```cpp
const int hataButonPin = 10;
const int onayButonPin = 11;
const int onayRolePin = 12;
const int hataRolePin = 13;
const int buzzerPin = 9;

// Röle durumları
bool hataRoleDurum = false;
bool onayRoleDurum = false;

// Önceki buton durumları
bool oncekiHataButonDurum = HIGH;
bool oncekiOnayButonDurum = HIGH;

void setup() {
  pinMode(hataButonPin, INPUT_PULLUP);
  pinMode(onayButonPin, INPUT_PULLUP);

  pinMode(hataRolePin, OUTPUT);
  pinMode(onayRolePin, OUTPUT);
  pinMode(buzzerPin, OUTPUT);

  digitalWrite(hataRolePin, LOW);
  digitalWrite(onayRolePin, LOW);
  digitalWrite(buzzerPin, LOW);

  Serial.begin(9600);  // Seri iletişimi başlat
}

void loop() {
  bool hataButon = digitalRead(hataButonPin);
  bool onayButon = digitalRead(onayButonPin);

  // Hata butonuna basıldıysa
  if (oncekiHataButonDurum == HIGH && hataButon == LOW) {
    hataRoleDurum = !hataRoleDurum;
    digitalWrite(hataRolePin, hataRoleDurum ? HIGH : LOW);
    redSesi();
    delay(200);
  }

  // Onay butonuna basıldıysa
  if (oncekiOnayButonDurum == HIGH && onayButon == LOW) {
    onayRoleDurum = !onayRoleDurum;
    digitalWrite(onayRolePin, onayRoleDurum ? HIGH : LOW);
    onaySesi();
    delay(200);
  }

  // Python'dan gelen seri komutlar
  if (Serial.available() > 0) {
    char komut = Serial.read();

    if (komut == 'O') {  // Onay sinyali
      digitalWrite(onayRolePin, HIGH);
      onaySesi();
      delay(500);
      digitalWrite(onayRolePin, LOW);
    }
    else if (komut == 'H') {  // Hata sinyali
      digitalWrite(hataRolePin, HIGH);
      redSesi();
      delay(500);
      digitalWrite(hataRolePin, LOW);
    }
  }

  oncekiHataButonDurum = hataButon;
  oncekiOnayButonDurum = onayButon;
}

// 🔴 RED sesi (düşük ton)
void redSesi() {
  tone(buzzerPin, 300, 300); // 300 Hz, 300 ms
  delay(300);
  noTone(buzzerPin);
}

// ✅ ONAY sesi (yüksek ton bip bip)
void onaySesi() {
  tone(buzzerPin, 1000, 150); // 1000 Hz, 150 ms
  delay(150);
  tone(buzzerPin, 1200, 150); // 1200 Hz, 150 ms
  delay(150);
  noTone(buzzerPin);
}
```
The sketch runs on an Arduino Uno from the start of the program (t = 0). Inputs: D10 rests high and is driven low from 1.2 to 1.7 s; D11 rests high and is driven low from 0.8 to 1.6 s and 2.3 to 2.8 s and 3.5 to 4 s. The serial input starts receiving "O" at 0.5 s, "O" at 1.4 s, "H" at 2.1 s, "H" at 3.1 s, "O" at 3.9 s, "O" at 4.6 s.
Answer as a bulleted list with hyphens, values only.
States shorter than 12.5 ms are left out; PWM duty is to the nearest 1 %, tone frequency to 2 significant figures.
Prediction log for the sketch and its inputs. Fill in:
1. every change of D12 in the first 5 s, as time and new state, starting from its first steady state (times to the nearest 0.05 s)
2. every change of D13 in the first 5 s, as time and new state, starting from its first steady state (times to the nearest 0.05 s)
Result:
- 0 s low; 0.5 s high; 1.3 s low; 1.8 s high; 3.1 s low
- 0 s low; 1.3 s high; 3.9 s low; 4.4 s high
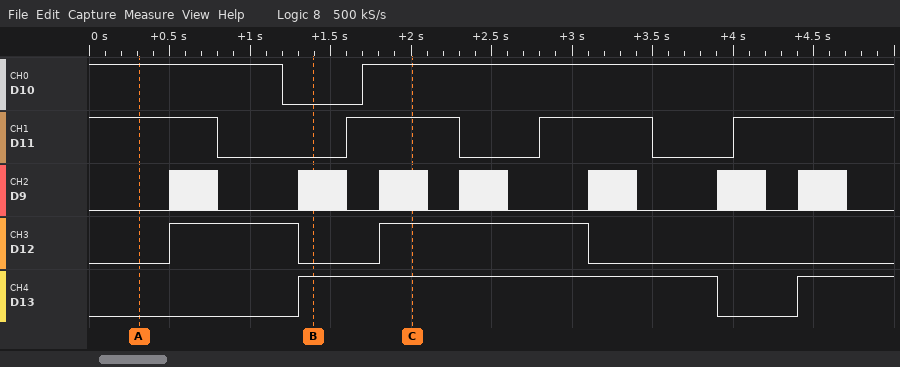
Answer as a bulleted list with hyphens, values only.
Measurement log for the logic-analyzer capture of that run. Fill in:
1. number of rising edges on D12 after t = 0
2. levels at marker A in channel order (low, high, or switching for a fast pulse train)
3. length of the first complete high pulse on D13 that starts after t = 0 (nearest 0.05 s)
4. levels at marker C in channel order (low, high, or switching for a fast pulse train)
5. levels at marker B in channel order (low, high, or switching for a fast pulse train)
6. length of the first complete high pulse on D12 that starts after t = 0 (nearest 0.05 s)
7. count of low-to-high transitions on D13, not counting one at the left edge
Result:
- 2
- D10 high, D11 high, D9 low, D12 low, D13 low
- 2.60 s
- D10 high, D11 high, D9 switching, D12 high, D13 high
- D10 low, D11 low, D9 switching, D12 low, D13 high
- 0.80 s
- 2
